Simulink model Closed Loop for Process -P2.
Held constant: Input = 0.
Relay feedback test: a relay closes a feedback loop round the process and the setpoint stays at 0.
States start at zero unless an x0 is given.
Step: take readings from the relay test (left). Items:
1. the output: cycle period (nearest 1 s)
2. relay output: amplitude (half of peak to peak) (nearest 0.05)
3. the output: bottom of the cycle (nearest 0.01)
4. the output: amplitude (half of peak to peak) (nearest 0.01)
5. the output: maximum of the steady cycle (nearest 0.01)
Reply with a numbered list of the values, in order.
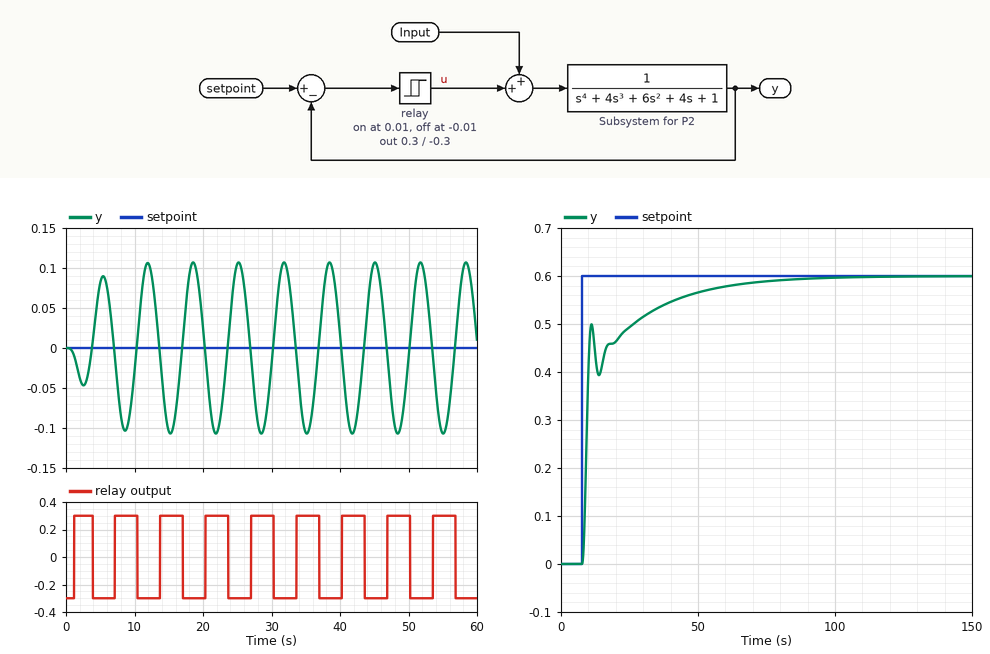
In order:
1. 7 s
2. 0.30
3. -0.11
4. 0.11
5. 0.11
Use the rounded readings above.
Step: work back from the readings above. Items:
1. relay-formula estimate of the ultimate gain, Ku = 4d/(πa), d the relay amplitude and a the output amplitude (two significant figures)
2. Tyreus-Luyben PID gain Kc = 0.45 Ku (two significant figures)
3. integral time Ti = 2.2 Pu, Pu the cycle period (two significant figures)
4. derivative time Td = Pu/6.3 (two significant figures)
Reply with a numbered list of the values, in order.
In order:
1. 3.5
2. 1.6
3. 15 s
4. 1.1 s
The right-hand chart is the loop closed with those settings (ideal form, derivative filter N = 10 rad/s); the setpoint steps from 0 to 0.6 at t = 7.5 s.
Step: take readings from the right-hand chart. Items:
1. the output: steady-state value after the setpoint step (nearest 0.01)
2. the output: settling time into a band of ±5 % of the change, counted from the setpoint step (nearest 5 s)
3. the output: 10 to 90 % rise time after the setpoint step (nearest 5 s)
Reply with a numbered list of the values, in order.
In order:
1. 0.60
2. 45 s
3. 30 s
